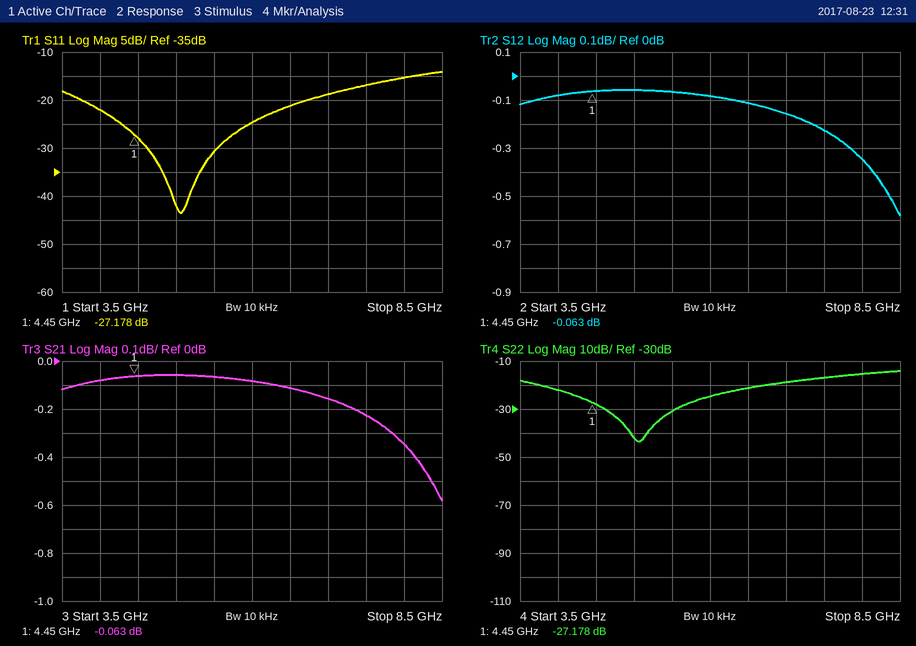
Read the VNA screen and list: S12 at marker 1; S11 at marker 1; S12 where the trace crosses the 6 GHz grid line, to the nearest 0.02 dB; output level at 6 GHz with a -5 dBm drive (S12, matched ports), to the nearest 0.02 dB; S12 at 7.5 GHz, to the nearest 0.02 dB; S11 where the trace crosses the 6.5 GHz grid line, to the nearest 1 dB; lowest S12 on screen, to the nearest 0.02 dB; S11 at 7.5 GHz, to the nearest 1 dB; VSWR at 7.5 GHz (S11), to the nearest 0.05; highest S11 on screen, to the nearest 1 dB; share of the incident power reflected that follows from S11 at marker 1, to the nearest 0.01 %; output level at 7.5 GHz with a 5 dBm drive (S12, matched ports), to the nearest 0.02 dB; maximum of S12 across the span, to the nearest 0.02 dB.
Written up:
-0.063 dB
-27.178 dB
-0.08 dB
-5.08 dBm
-0.22 dB
-21 dB
-0.58 dB
-17 dB
1.35
-14 dB
0.19 %
4.78 dBm
-0.06 dB
